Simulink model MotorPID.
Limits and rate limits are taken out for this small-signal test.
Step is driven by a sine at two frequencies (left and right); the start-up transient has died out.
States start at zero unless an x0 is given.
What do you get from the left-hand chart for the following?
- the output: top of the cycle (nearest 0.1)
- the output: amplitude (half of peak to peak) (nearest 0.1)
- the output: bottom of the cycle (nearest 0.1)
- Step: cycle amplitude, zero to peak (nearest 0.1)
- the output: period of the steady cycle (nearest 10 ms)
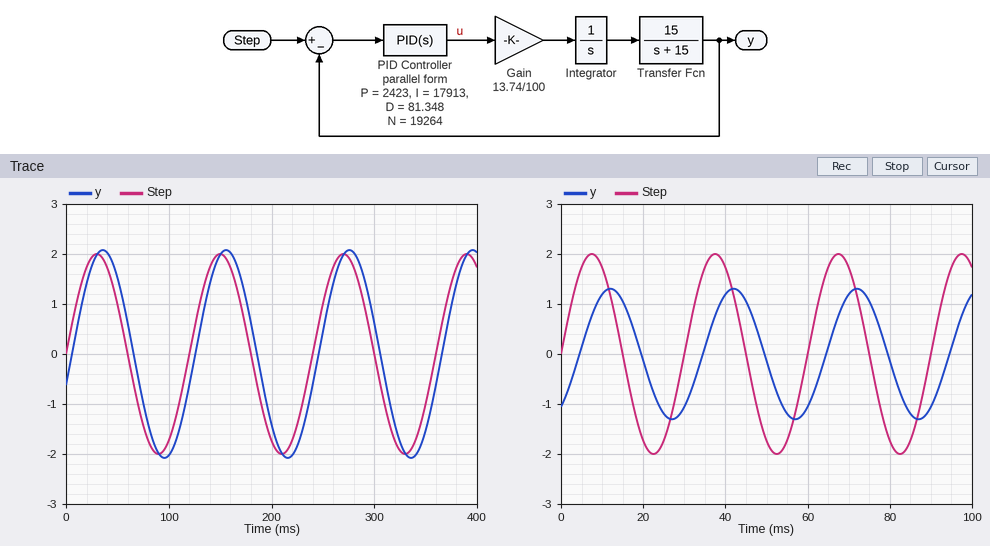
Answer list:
2.1
2.1
-2.1
2.0
120 ms
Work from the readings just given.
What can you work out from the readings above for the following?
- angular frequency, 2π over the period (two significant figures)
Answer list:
0.052 rad/ms
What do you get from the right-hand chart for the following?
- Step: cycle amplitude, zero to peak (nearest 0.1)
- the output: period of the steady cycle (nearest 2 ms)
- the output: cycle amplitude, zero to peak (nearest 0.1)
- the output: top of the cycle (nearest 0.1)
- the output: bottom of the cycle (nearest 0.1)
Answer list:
2.0
30 ms
1.3
1.3
-1.3
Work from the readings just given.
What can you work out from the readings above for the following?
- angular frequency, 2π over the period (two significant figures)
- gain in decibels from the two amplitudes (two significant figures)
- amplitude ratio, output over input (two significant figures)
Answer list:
0.21 rad/ms
-3.7 dB
0.65
